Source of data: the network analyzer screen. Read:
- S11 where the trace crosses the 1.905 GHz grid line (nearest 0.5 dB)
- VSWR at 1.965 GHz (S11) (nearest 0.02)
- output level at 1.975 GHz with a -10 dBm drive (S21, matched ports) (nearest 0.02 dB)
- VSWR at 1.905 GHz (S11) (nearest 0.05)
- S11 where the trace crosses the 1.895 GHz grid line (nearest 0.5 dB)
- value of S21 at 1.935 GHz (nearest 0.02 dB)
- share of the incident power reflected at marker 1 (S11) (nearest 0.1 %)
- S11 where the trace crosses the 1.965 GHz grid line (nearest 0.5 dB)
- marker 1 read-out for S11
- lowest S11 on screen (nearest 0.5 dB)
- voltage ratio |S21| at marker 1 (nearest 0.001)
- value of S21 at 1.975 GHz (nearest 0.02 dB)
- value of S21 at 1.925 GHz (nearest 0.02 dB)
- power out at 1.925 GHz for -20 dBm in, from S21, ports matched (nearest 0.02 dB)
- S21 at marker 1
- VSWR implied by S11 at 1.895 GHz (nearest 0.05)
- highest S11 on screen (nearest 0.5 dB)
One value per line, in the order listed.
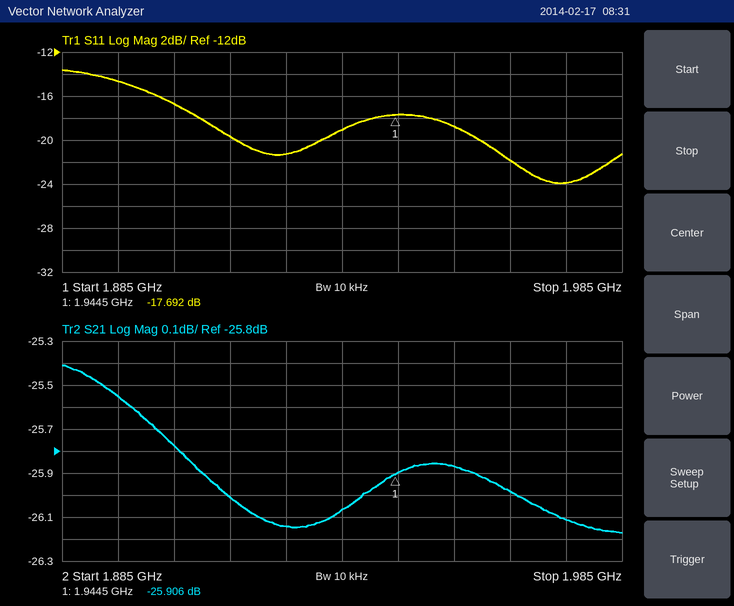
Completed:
-16.5 dB
1.18
-36.12 dBm
1.35
-14.5 dB
-26.06 dB
1.7 %
-22.0 dB
-17.692 dB
-24.0 dB
0.051
-26.12 dB
-26.14 dB
-46.14 dBm
-25.906 dB
1.45
-13.5 dB
